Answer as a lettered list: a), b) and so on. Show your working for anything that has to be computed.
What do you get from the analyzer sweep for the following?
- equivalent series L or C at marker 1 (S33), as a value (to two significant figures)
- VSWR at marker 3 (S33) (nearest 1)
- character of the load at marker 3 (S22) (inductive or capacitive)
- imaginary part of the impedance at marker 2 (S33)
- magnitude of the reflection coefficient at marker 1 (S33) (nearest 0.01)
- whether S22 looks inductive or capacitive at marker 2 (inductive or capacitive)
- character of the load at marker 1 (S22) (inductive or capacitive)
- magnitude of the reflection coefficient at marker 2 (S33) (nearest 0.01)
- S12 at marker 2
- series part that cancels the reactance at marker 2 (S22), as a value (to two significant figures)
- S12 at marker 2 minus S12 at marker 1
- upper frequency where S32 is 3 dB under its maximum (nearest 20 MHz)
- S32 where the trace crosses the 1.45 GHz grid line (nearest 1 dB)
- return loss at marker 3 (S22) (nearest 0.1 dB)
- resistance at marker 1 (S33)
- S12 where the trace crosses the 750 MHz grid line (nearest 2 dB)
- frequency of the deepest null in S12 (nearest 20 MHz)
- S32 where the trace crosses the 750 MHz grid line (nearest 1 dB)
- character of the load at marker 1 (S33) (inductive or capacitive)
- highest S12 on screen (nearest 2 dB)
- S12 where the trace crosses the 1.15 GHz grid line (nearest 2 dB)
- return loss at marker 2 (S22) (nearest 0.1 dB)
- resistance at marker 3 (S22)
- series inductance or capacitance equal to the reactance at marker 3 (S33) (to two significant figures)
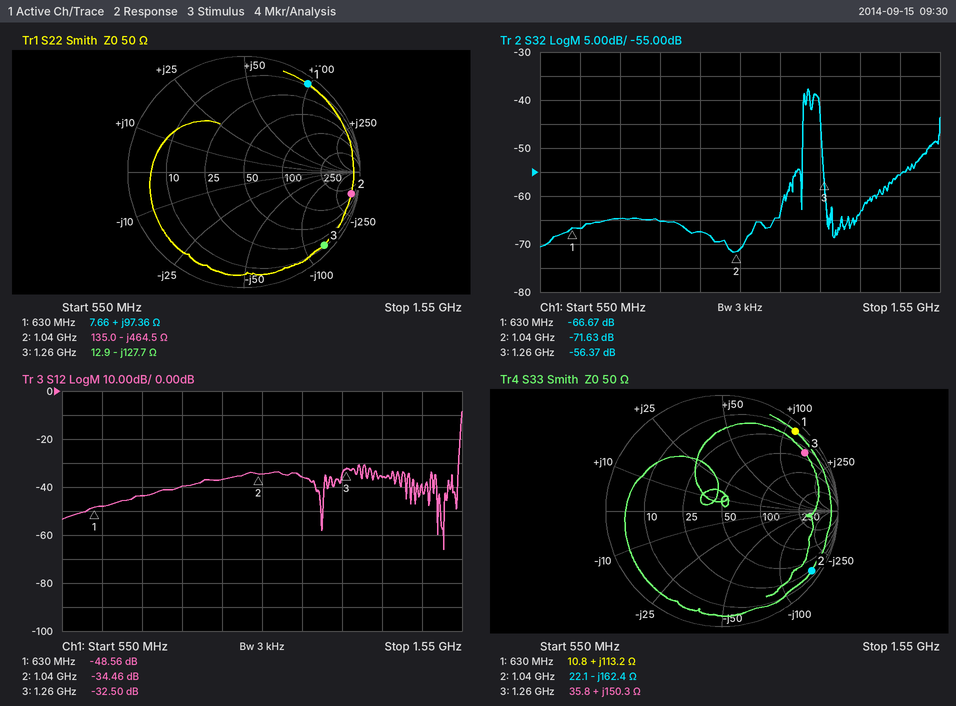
a) L = 113.2 Ω/(2π × 630 MHz) ≈ 29 nH
b) 15
c) capacitive
d) -162.4 Ω
e) 0.93
f) capacitive
g) inductive
h) 0.93
i) -34.46 dB
j) L = 464.5 Ω/(2π × 1.04 GHz) ≈ 71 nH
k) -34.46 − (-48.56) = 14.10 dB
l) 1.22 GHz
m) -56 dB
n) 0.6 dB
o) 10.8 Ω
p) -44 dB
q) 1.50 GHz
r) -65 dB
s) inductive
t) -8 dB
u) -36 dB
v) 0.5 dB
w) 12.9 Ω
x) L = 150.3 Ω/(2π × 1.26 GHz) ≈ 19 nH
